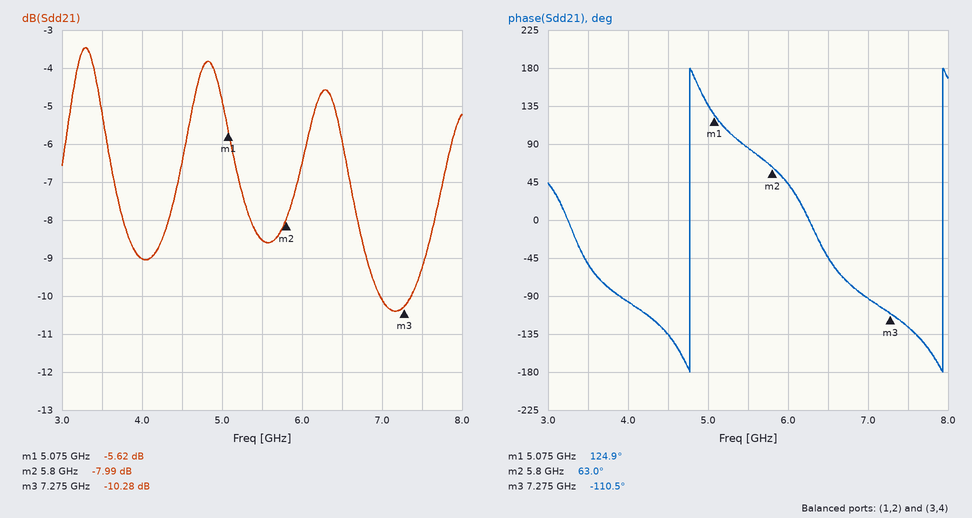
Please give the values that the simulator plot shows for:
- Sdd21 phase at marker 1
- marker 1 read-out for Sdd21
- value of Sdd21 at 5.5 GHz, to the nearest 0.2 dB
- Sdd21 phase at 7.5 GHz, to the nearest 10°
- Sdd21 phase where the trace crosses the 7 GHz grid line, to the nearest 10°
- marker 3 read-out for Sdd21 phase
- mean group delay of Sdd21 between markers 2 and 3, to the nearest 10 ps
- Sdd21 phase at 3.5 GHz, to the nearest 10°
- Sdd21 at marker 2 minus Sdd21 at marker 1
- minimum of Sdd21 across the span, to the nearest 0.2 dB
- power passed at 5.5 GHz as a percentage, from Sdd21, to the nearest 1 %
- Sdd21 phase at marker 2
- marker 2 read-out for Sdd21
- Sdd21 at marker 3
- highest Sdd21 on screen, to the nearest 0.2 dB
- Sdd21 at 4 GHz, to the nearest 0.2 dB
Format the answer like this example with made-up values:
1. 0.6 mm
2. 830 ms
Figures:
1. 124.9°
2. -5.62 dB
3. -8.6 dB
4. -130°
5. -90°
6. -110.5°
7. 330 ps
8. -50°
9. -2.37 dB
10. -10.4 dB
11. 14 %
12. 63.0°
13. -7.99 dB
14. -10.28 dB
15. -3.4 dB
16. -9.0 dB
